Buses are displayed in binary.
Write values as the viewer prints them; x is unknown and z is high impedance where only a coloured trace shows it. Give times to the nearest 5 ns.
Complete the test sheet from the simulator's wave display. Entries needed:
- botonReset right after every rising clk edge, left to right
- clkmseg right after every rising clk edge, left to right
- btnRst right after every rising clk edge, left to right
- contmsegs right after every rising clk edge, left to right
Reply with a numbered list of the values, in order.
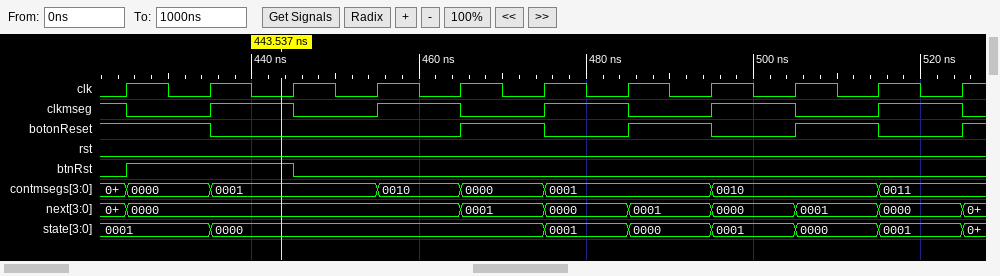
1. 1 0 0 0 1 0 1 0 1 0 1
2. 0 1 0 1 0 1 0 1 0 1 0
3. 1 1 0 0 0 0 0 0 0 0 0
4. 0000, 0001, 0001, 0010, 0000, 0001, 0001, 0010, 0010, 0011, 0011
